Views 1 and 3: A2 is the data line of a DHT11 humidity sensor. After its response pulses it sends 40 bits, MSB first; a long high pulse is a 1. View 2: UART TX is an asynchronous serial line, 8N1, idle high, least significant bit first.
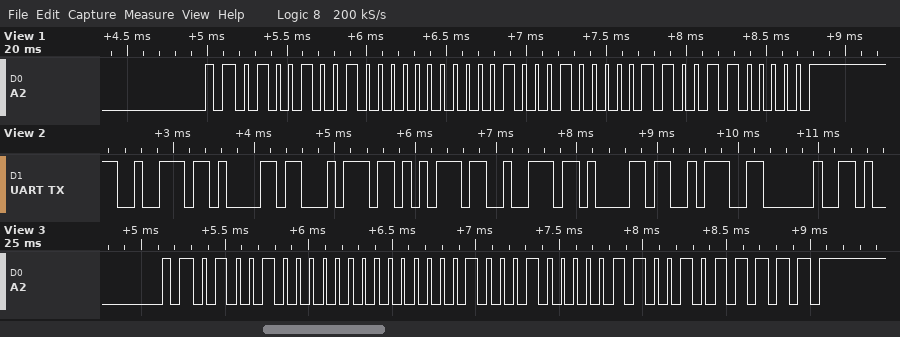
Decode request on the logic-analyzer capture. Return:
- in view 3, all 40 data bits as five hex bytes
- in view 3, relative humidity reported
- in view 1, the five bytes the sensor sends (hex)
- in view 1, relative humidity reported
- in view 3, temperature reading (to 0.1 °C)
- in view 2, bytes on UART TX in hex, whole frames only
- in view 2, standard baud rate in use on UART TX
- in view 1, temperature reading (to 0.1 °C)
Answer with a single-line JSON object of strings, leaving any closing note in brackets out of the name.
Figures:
{"in view 3, all 40 data bits as five hex bytes": "48 00 11 06 5F", "in view 3, relative humidity reported": "72 %", "in view 1, the five bytes the sensor sends": "49 00 11 06 60", "in view 1, relative humidity reported": "73 %", "in view 3, temperature reading": "17.6 °C", "in view 2, bytes on UART TX in hex, whole frames only": "0x72 0x61 0x74 0x75 0x72 0x61 0x3A 0x20", "in view 2, standard baud rate in use on UART TX": "9600 baud", "in view 1, temperature reading": "17.6 °C"}
